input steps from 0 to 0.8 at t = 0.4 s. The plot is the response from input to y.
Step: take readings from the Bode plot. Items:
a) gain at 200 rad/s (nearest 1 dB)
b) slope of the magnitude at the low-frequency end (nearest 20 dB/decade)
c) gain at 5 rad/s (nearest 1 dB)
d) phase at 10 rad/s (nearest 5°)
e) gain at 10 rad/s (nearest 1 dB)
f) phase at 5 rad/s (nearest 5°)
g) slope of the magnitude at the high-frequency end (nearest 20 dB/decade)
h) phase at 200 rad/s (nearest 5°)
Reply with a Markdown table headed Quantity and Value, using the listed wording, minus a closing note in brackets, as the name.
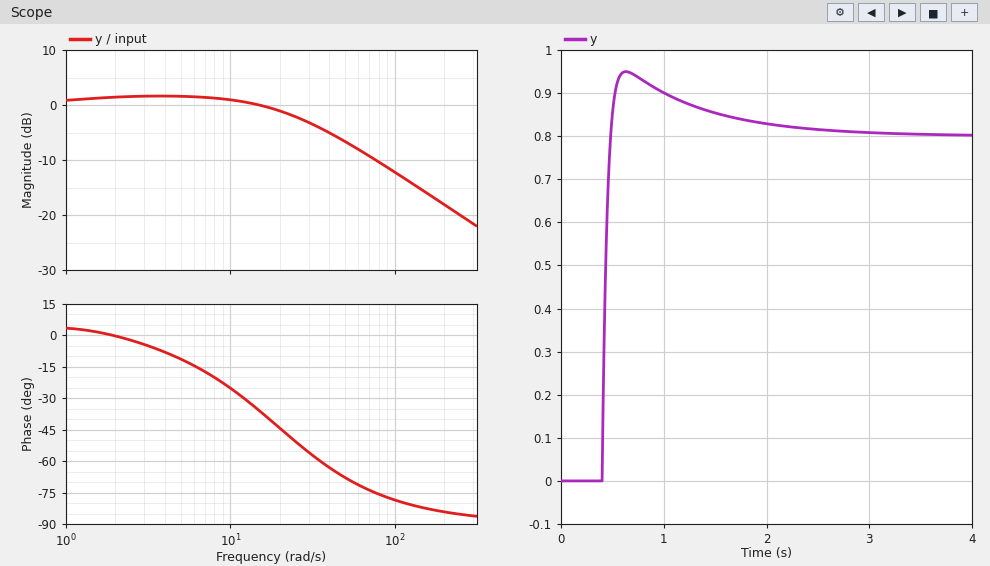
| Quantity | Value |
|---|---|
| gain at 200 rad/s | -18 dB |
| slope of the magnitude at the low-frequency end | 0 dB/decade |
| gain at 5 rad/s | 2 dB |
| phase at 10 rad/s | -25° |
| gain at 10 rad/s | 1 dB |
| phase at 5 rad/s | -10° |
| slope of the magnitude at the high-frequency end | -20 dB/decade |
| phase at 200 rad/s | -85° |
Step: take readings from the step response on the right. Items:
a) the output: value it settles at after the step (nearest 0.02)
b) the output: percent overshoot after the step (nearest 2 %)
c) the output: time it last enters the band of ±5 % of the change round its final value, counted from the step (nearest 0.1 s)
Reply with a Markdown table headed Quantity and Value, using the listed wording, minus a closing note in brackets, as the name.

| Quantity | Value |
|---|---|
| the output: value it settles at after the step | 0.80 |
| the output: percent overshoot after the step | 18 % |
| the output: time it last enters the band of ±5 % of the change round its final value, counted from the step | 1.3 s |
